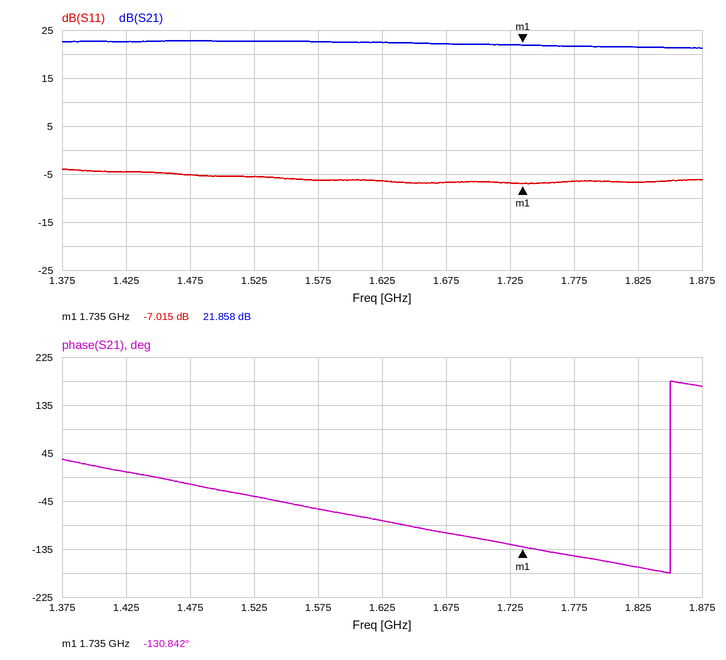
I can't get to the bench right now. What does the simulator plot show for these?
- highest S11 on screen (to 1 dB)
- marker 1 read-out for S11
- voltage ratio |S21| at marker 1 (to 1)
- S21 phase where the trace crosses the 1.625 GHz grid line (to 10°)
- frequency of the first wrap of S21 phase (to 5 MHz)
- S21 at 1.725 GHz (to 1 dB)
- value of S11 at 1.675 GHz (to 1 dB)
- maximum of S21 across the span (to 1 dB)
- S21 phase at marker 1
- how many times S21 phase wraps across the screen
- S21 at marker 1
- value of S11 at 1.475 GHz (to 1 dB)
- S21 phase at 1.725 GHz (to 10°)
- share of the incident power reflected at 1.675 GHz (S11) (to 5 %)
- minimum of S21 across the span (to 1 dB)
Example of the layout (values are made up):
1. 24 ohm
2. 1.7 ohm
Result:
1. -4 dB
2. -7.015 dB
3. 12
4. -80°
5. 1.850 GHz
6. 22 dB
7. -7 dB
8. 23 dB
9. -130.842°
10. 1
11. 21.858 dB
12. -5 dB
13. -130°
14. 20 %
15. 21 dB
